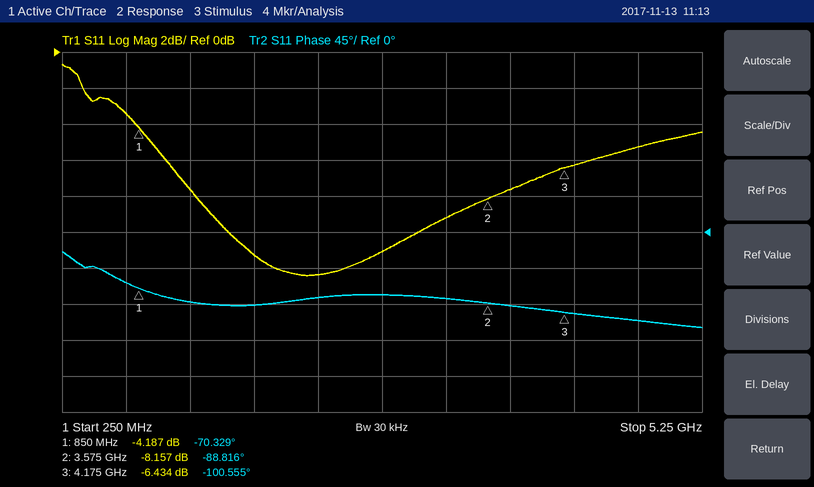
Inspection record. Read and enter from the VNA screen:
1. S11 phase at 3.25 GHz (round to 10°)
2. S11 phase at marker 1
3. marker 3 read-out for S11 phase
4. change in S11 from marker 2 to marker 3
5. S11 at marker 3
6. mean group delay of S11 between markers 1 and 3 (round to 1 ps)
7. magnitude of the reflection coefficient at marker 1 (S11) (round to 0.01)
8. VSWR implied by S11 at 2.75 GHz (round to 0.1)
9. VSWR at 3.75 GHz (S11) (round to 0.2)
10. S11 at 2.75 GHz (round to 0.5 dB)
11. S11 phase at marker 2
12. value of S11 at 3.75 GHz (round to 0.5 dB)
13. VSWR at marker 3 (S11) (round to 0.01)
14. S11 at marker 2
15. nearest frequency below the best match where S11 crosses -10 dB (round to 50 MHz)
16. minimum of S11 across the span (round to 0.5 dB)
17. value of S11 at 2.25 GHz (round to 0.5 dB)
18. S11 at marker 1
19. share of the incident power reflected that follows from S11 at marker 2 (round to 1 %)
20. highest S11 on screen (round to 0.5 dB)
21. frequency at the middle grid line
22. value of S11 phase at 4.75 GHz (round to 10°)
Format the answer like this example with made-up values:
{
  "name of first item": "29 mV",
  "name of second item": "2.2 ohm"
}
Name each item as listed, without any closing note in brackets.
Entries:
{
  "S11 phase at 3.25 GHz": "-80°",
  "S11 phase at marker 1": "-70.329°",
  "marker 3 read-out for S11 phase": "-100.555°",
  "change in S11 from marker 2 to marker 3": "1.723 dB",
  "S11 at marker 3": "-6.434 dB",
  "mean group delay of S11 between markers 1 and 3": "25 ps",
  "magnitude of the reflection coefficient at marker 1 (S11)": "0.62",
  "VSWR implied by S11 at 2.75 GHz": "1.8",
  "VSWR at 3.75 GHz (S11)": "2.4",
  "S11 at 2.75 GHz": "-11.0 dB",
  "S11 phase at marker 2": "-88.816°",
  "value of S11 at 3.75 GHz": "-7.5 dB",
  "VSWR at marker 3 (S11)": "2.82",
  "S11 at marker 2": "-8.157 dB",
  "nearest frequency below the best match where S11 crosses -10 dB": "1.55 GHz",
  "minimum of S11 across the span": "-12.5 dB",
  "value of S11 at 2.25 GHz": "-12.5 dB",
  "S11 at marker 1": "-4.187 dB",
  "share of the incident power reflected that follows from S11 at marker 2": "15 %",
  "highest S11 on screen": "-0.5 dB",
  "frequency at the middle grid line": "2.75 GHz",
  "value of S11 phase at 4.75 GHz": "-110°"
}
